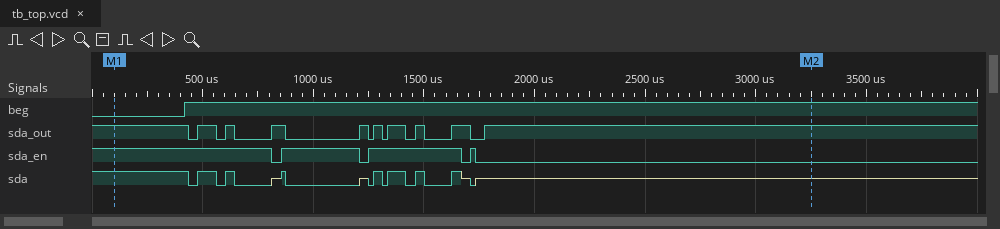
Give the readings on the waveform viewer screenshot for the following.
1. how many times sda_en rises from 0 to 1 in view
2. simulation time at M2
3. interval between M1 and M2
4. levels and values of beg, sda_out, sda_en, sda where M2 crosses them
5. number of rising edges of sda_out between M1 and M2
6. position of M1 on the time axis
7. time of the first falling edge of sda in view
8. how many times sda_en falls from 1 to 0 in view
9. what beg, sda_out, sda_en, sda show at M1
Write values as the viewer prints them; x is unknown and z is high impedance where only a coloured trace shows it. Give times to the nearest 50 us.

3
3250 us
3150 us
beg=1, sda_out=1, sda_en=0, sda=z
9
100 us
450 us
4
beg=0, sda_out=1, sda_en=1, sda=1
